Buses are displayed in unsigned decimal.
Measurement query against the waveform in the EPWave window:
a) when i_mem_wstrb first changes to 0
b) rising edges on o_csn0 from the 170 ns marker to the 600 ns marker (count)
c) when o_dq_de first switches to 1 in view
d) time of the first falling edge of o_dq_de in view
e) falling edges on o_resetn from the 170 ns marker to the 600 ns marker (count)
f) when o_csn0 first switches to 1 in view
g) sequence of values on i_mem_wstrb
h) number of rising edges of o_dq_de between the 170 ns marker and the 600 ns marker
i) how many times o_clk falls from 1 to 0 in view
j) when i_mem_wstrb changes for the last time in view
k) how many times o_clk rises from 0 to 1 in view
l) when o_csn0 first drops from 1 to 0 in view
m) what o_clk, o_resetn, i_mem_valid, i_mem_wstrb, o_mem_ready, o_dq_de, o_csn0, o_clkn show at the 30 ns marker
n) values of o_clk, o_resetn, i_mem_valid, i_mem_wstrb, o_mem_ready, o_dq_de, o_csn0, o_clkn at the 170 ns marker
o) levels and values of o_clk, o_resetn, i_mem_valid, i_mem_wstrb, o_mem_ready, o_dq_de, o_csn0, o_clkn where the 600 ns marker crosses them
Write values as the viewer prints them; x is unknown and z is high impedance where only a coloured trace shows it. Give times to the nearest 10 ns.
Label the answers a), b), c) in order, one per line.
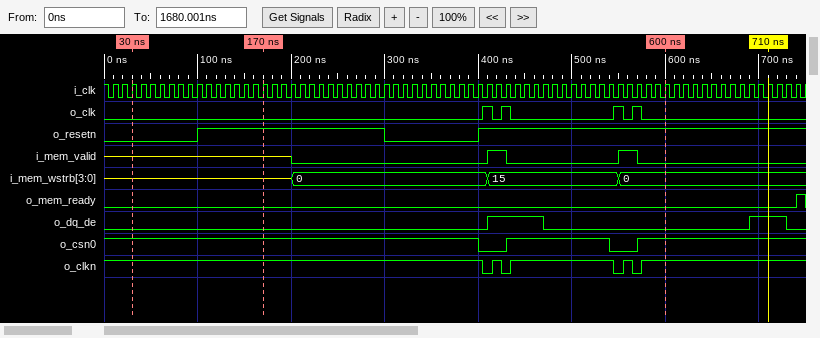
a) 200 ns
b) 2
c) 410 ns
d) 470 ns
e) 1
f) 430 ns
g) z, 0, 15, 0
h) 1
i) 4
j) 550 ns
k) 4
l) 400 ns
m) o_clk=0, o_resetn=0, i_mem_valid=z, i_mem_wstrb=z, o_mem_ready=0, o_dq_de=0, o_csn0=1, o_clkn=1
n) o_clk=0, o_resetn=1, i_mem_valid=z, i_mem_wstrb=z, o_mem_ready=0, o_dq_de=0, o_csn0=1, o_clkn=1
o) o_clk=0, o_resetn=1, i_mem_valid=0, i_mem_wstrb=0, o_mem_ready=0, o_dq_de=0, o_csn0=1, o_clkn=1
